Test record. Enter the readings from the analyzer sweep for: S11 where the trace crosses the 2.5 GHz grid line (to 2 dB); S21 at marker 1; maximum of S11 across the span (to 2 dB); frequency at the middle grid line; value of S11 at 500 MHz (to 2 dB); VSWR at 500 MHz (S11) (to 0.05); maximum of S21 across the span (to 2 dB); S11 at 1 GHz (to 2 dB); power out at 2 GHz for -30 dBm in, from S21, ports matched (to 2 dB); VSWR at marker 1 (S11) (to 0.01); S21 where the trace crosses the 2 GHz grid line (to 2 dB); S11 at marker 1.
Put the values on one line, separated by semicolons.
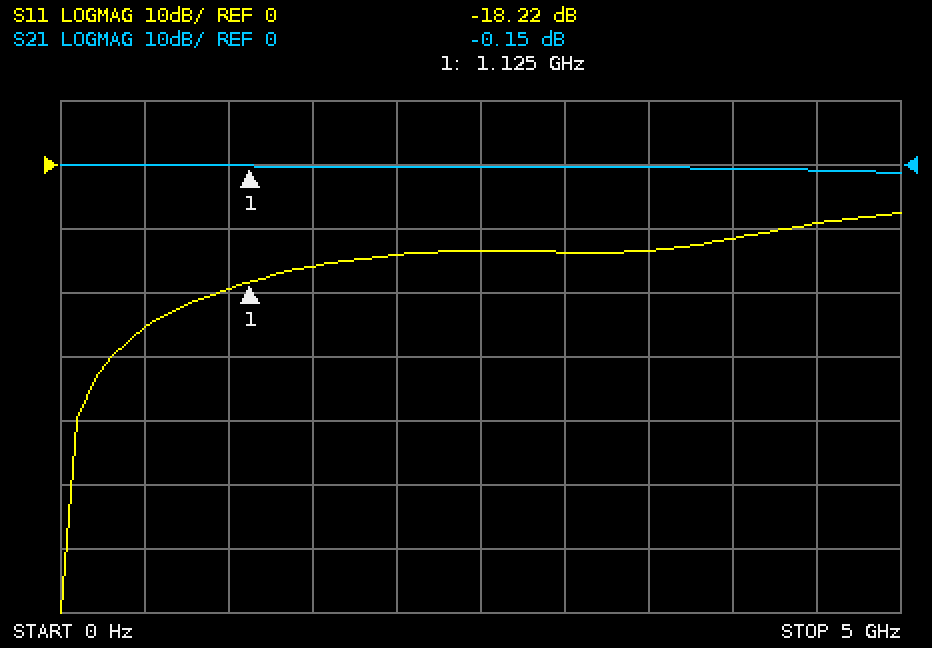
-14 dB; -0.15 dB; -8 dB; 2.5 GHz; -26 dB; 1.10; 0 dB; -20 dB; -30 dBm; 1.28; 0 dB; -18.22 dB
